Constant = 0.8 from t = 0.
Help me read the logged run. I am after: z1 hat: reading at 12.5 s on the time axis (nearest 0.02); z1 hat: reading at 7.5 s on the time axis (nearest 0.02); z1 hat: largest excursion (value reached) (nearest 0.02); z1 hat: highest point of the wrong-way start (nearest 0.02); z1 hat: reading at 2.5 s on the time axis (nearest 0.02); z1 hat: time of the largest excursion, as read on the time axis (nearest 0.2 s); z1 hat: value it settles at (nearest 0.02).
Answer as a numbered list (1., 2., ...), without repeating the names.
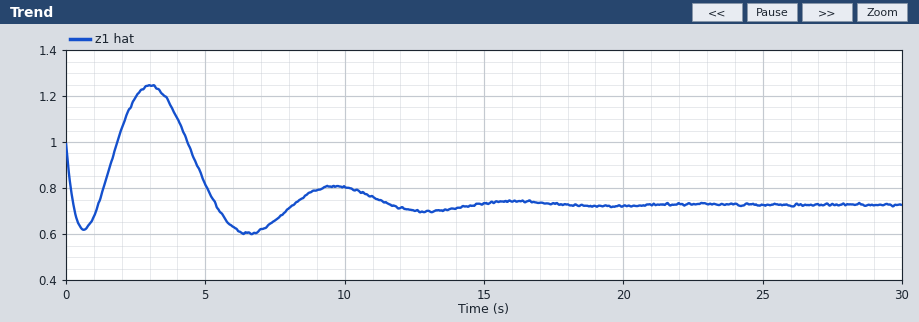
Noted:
1. 0.70
2. 0.66
3. 0.60
4. 1.24
5. 1.20
6. 6.6 s
7. 0.72
